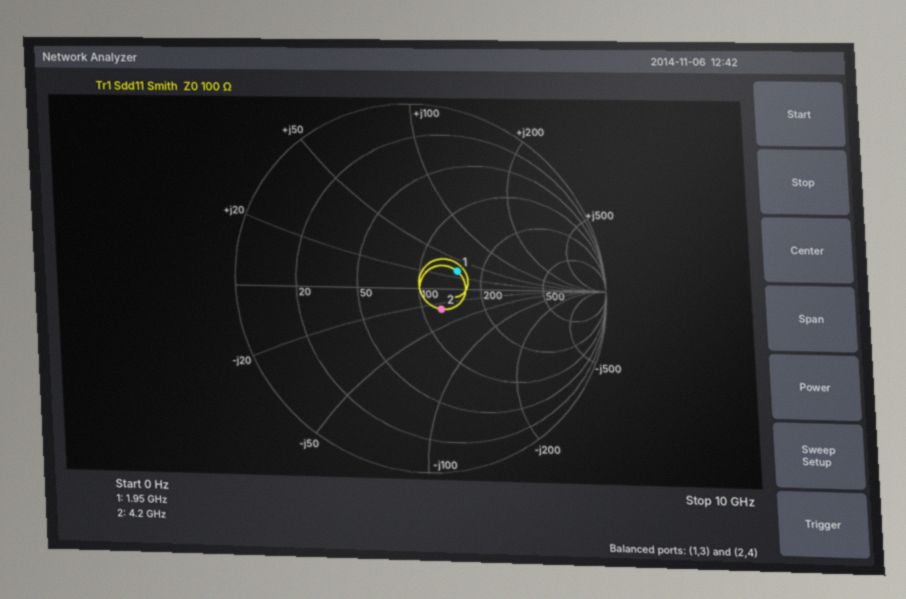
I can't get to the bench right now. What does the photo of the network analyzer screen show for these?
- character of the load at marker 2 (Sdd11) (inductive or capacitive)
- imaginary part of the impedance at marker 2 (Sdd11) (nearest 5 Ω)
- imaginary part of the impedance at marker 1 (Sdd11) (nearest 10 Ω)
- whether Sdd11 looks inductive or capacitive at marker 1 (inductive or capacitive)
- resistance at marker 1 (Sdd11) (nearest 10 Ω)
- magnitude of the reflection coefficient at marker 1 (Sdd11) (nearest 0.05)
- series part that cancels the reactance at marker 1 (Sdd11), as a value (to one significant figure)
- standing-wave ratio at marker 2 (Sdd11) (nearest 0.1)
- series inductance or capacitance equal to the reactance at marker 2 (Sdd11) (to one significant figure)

capacitive
-30 Ω
+30 Ω
inductive
150 Ω
0.25
3 pF
1.4
1 pF
